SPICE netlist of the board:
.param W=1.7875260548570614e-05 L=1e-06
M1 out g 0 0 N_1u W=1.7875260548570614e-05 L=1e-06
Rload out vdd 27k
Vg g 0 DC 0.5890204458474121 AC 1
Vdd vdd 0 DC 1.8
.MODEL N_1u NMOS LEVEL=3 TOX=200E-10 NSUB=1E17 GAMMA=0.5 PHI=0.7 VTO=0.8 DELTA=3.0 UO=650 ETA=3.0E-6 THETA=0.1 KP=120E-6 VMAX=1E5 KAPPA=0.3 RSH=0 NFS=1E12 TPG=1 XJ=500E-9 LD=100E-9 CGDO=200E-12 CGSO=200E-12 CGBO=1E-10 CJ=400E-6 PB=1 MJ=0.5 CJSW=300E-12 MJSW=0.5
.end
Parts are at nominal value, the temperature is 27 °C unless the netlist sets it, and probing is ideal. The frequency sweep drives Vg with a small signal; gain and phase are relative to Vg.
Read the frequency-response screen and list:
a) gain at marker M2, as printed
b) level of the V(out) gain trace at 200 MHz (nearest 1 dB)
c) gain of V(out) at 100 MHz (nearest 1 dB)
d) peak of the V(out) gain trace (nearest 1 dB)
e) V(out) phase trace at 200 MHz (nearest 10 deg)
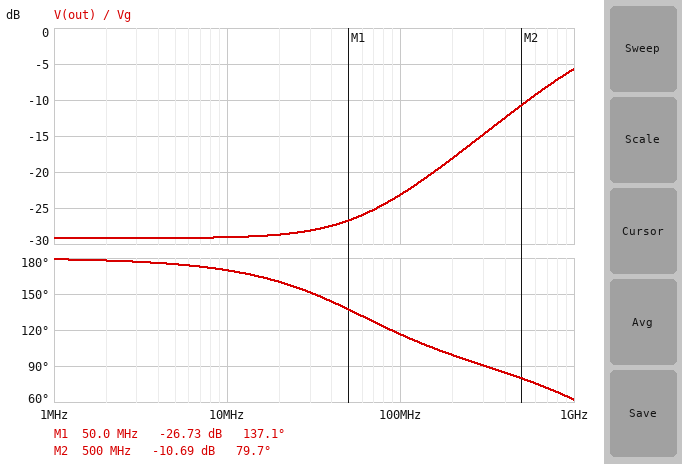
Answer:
-10.69 dB
-18 dB
-23 dB
-6 dB
100 deg
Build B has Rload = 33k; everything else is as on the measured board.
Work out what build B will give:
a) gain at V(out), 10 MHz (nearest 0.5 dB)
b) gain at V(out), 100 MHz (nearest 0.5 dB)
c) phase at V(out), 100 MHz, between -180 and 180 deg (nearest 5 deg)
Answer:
-27.5 dB
-21.5 dB
115 deg
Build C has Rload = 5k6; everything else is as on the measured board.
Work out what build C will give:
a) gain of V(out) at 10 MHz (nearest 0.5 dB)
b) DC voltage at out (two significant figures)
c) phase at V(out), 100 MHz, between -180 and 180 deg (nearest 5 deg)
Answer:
-42.5 dB
1.8 V
120 deg
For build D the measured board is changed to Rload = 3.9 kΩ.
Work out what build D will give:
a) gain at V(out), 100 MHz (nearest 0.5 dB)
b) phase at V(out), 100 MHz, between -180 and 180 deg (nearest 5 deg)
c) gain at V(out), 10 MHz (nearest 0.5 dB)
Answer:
-40.0 dB
120 deg
-46.0 dB
